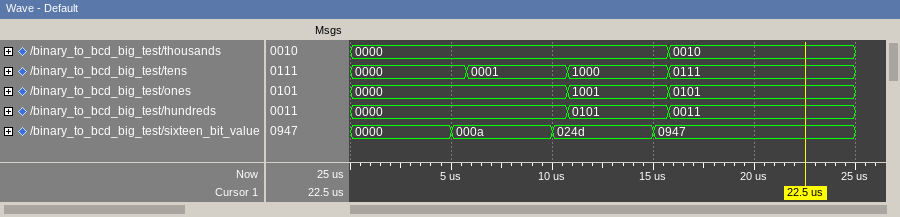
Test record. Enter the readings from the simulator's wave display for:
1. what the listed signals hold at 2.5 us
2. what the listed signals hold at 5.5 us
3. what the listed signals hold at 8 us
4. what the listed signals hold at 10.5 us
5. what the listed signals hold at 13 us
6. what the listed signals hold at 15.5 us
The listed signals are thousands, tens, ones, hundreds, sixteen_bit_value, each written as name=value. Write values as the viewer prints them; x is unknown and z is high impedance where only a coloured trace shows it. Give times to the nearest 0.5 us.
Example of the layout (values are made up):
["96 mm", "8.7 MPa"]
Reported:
["thousands=0000, tens=0000, ones=0000, hundreds=0000, sixteen_bit_value=0000", "thousands=0000, tens=0000, ones=0000, hundreds=0000, sixteen_bit_value=000a", "thousands=0000, tens=0001, ones=0000, hundreds=0000, sixteen_bit_value=000a", "thousands=0000, tens=0001, ones=0000, hundreds=0000, sixteen_bit_value=024d", "thousands=0000, tens=1000, ones=1001, hundreds=0101, sixteen_bit_value=024d", "thousands=0000, tens=1000, ones=1001, hundreds=0101, sixteen_bit_value=0947"]
